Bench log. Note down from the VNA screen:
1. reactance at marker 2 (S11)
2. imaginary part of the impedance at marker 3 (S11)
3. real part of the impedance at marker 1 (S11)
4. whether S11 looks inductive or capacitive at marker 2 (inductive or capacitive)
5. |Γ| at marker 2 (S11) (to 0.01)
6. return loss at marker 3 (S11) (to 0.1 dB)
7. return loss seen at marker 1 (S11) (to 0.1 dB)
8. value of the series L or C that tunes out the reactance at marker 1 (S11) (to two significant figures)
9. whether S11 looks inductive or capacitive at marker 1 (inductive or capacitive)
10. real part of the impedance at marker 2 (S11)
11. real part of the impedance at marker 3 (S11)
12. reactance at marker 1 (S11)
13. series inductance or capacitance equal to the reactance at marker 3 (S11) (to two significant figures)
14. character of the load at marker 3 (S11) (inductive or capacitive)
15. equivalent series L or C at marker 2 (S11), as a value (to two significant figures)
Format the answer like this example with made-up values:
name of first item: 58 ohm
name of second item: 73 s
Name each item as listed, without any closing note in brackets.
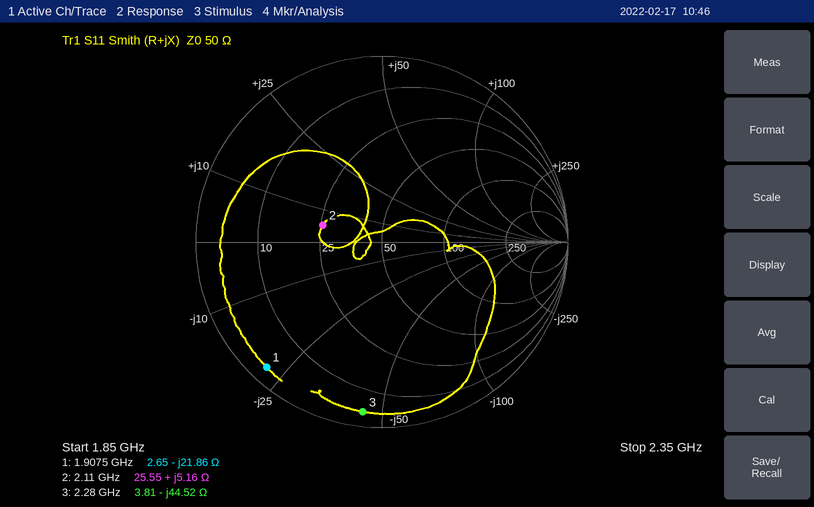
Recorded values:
reactance at marker 2: +5.16 Ω
imaginary part of the impedance at marker 3: -44.52 Ω
real part of the impedance at marker 1: 2.65 Ω
whether S11 looks inductive or capacitive at marker 2: inductive
|Γ| at marker 2 (S11): 0.33
return loss at marker 3 (S11): 0.7 dB
return loss seen at marker 1 (S11): 0.8 dB
value of the series L or C that tunes out the reactance at marker 1 (S11): 1.8 nH
whether S11 looks inductive or capacitive at marker 1: capacitive
real part of the impedance at marker 2: 25.55 Ω
real part of the impedance at marker 3: 3.81 Ω
reactance at marker 1: -21.86 Ω
series inductance or capacitance equal to the reactance at marker 3 (S11): 1.6 pF
character of the load at marker 3 (S11): capacitive
equivalent series L or C at marker 2 (S11), as a value: 390 pH
